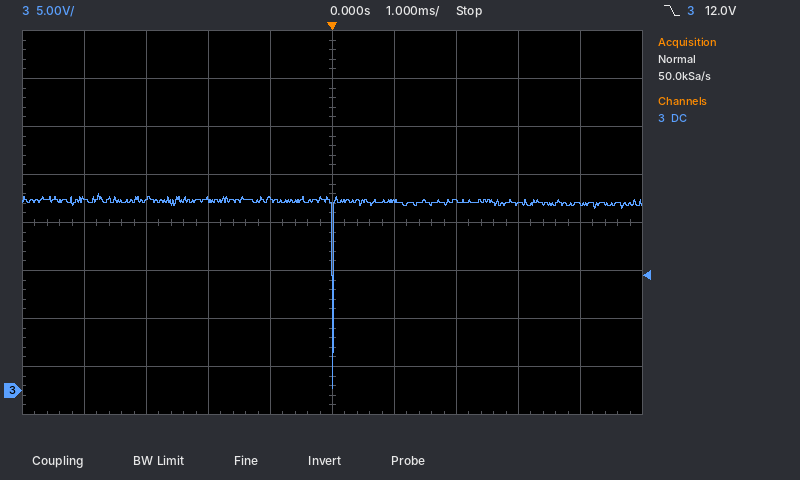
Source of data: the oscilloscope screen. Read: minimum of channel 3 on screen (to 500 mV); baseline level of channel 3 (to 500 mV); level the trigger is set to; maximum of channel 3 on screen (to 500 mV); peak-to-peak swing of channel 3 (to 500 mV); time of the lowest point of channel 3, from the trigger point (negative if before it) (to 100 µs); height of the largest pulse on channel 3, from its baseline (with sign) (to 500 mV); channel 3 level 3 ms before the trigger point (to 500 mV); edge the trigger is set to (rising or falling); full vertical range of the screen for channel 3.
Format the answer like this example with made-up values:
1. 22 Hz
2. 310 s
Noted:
1. 0.0 V
2. 19.5 V
3. 12.0 V
4. 20.5 V
5. 20.5 V
6. 0.0 ms
7. -19.5 V
8. 20.0 V
9. falling
10. 40 V
